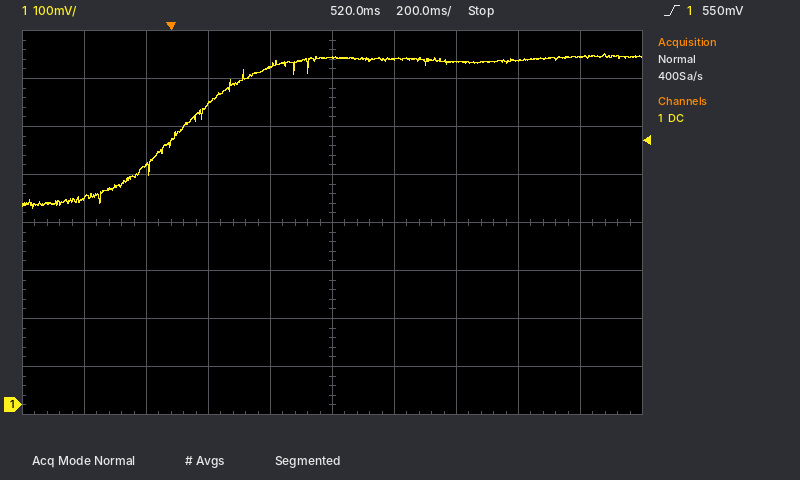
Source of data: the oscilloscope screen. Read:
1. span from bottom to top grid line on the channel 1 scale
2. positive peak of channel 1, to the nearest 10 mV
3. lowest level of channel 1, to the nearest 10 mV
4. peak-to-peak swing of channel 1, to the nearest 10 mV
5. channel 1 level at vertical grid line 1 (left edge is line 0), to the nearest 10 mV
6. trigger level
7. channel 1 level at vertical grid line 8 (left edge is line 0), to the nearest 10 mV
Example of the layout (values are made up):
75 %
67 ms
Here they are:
800 mV
730 mV
410 mV
320 mV
430 mV
550 mV
720 mV
